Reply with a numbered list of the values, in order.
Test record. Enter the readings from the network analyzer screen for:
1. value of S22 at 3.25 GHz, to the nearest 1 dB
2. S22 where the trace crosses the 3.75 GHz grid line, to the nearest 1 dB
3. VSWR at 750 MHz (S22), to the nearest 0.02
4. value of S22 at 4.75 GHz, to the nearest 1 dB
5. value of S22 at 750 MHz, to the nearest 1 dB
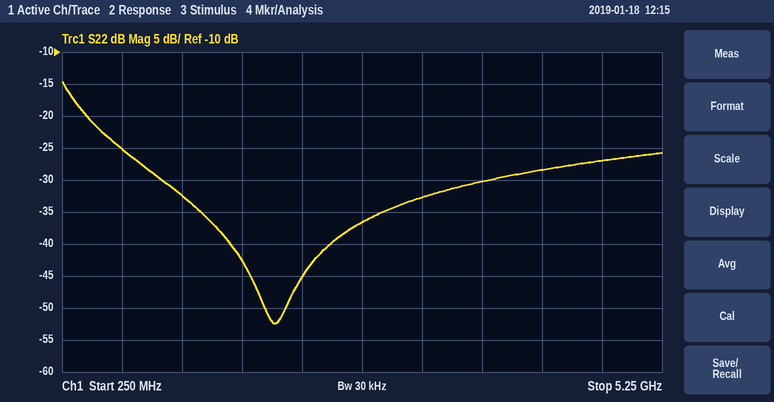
1. -33 dB
2. -30 dB
3. 1.12
4. -27 dB
5. -25 dB
